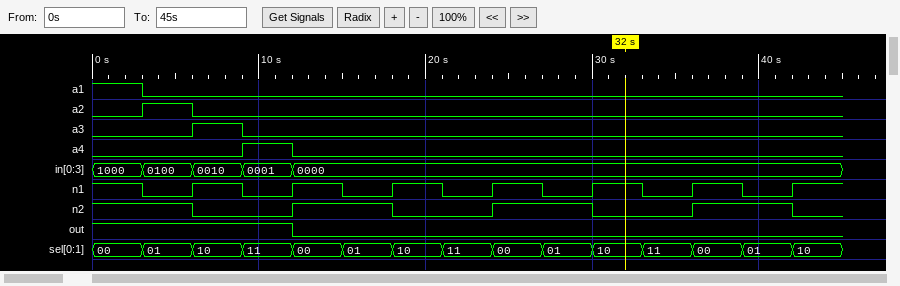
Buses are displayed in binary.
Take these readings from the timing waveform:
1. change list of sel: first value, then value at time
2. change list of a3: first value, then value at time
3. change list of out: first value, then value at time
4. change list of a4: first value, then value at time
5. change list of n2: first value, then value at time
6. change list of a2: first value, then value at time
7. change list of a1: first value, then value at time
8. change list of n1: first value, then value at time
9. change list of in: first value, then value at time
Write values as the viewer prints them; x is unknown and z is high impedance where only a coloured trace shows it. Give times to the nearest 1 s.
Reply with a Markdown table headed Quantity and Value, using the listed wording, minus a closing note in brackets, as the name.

| Quantity | Value |
|---|---|
| change list of sel: first value, then value at time | 00, 01 at 3 s, 10 at 6 s, 11 at 9 s, 00 at 12 s, 01 at 15 s, 10 at 18 s, 11 at 21 s, 00 at 24 s, 01 at 27 s, 10 at 30 s, 11 at 33 s, 00 at 36 s, 01 at 39 s, 10 at 42 s |
| change list of a3: first value, then value at time | 0, 1 at 6 s, 0 at 9 s |
| change list of out: first value, then value at time | 1, 0 at 12 s |
| change list of a4: first value, then value at time | 0, 1 at 9 s, 0 at 12 s |
| change list of n2: first value, then value at time | 1, 0 at 6 s, 1 at 12 s, 0 at 18 s, 1 at 24 s, 0 at 30 s, 1 at 36 s, 0 at 42 s |
| change list of a2: first value, then value at time | 0, 1 at 3 s, 0 at 6 s |
| change list of a1: first value, then value at time | 1, 0 at 3 s |
| change list of n1: first value, then value at time | 1, 0 at 3 s, 1 at 6 s, 0 at 9 s, 1 at 12 s, 0 at 15 s, 1 at 18 s, 0 at 21 s, 1 at 24 s, 0 at 27 s, 1 at 30 s, 0 at 33 s, 1 at 36 s, 0 at 39 s, 1 at 42 s |
| change list of in: first value, then value at time | 1000, 0100 at 3 s, 0010 at 6 s, 0001 at 9 s, 0000 at 12 s |
